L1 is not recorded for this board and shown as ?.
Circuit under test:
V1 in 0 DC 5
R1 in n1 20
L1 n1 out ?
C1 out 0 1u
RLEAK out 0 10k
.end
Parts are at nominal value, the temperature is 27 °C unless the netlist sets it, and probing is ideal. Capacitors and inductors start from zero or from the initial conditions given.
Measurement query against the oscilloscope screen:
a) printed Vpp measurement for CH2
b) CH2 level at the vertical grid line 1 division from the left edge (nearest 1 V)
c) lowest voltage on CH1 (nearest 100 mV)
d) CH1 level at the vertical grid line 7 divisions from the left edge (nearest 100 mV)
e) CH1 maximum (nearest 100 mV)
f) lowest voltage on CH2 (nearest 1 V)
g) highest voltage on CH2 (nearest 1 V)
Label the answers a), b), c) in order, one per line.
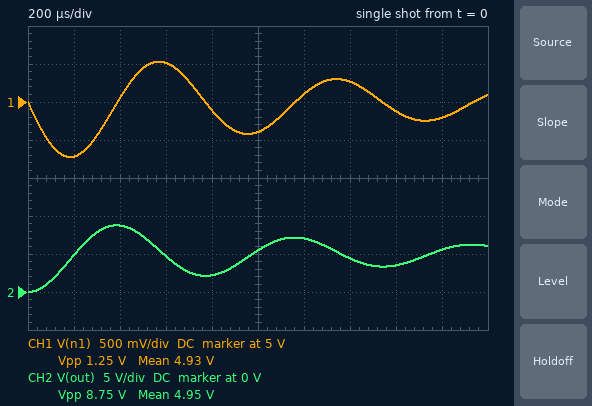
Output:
a) 8.75 V
b) 5 V
c) 4.3 V
d) 5.3 V
e) 5.5 V
f) 0 V
g) 9 V
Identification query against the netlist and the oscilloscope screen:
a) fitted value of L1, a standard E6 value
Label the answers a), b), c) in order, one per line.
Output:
a) 15 mH
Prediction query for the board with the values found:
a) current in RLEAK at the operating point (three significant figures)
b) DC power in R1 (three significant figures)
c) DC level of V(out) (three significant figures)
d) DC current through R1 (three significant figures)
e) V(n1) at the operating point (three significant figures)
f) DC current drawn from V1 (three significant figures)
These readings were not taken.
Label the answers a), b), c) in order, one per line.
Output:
a) 499 µA
b) 4.98 µW
c) 4.99 V
d) 499 µA
e) 4.99 V
f) 499 µA
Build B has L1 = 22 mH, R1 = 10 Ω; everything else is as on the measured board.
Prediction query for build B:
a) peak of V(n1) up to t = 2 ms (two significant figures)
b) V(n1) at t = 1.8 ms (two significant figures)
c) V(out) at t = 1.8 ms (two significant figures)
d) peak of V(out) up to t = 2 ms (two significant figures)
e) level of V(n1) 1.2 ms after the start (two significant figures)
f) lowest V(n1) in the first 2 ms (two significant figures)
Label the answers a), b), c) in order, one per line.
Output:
a) 5.3 V
b) 5.1 V
c) 2.3 V
d) 9.4 V
e) 4.8 V
f) 4.7 V
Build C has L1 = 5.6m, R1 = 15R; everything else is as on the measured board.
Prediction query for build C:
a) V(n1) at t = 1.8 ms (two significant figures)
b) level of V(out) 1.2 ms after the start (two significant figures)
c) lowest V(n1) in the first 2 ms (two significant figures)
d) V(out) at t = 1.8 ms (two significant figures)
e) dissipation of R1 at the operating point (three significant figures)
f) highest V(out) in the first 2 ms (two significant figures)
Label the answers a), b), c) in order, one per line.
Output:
a) 5.1 V
b) 5.9 V
c) 4.1 V
d) 4.9 V
e) 3.74 µW
f) 8.6 V
